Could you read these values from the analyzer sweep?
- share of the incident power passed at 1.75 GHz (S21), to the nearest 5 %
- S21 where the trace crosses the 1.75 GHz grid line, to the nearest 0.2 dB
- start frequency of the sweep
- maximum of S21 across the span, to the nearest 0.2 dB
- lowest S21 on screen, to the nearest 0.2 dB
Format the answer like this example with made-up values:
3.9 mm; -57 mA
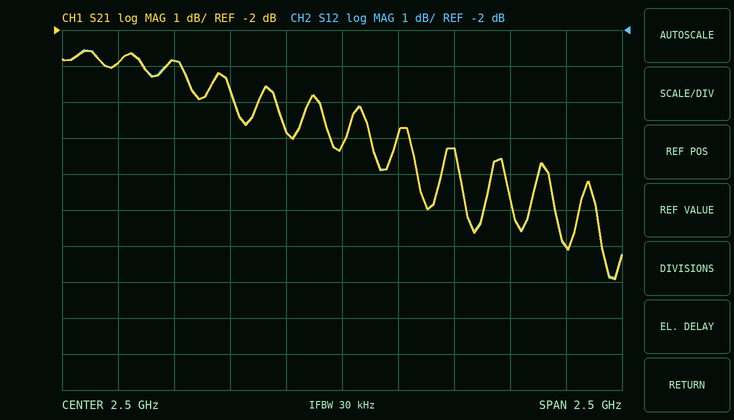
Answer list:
50 %; -2.8 dB; 1.25 GHz; -2.6 dB; -9.0 dB
